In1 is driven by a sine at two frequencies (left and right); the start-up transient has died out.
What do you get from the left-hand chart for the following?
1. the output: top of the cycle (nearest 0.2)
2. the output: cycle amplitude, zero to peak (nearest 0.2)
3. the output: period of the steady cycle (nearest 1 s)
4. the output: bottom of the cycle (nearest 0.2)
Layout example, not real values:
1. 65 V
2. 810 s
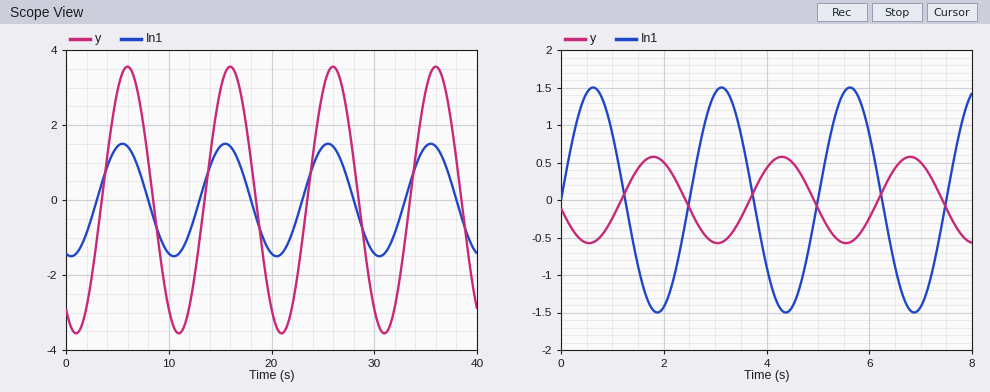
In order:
1. 3.6
2. 3.6
3. 10 s
4. -3.6
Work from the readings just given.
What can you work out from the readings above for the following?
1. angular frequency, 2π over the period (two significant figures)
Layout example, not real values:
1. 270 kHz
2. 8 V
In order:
1. 0.63 rad/s
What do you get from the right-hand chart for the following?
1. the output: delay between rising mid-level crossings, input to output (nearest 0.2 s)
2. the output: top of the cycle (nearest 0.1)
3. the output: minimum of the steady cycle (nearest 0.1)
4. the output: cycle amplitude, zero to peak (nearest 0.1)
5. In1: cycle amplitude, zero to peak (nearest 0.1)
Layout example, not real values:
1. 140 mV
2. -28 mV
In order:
1. 1.2 s
2. 0.6
3. -0.6
4. 0.6
5. 1.5
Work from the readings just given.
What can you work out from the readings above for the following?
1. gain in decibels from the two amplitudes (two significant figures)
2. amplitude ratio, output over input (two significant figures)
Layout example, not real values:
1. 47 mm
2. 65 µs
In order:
1. -8.0 dB
2. 0.40
